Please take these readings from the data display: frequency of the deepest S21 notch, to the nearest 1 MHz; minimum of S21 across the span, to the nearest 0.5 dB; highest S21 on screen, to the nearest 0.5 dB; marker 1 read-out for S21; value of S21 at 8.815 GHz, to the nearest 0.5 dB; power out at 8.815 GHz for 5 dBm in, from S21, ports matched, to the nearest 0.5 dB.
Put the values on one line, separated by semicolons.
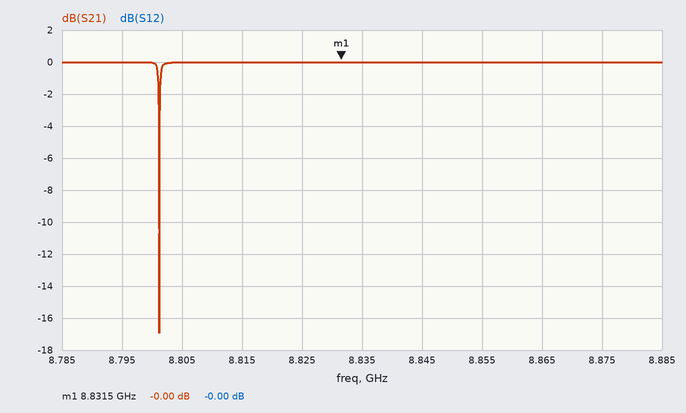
8.801 GHz; -17.0 dB; 0.0 dB; -0.00 dB; 0.0 dB; 5.0 dBm
